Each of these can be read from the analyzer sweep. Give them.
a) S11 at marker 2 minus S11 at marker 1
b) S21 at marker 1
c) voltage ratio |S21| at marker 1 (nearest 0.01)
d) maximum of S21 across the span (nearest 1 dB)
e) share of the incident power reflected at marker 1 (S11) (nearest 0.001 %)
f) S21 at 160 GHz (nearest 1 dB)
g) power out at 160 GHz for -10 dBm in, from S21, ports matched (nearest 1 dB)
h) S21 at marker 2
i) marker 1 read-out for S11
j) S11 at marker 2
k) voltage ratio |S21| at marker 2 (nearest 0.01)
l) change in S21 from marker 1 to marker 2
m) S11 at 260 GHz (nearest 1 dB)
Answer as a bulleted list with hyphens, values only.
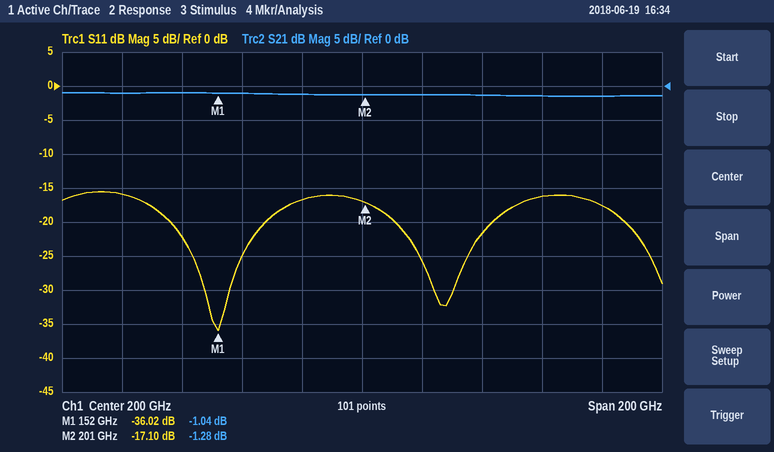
- 18.92 dB
- -1.04 dB
- 0.89
- -1 dB
- 0.025 %
- -1 dB
- -11 dBm
- -1.28 dB
- -36.02 dB
- -17.10 dB
- 0.86
- -0.24 dB
- -16 dB
